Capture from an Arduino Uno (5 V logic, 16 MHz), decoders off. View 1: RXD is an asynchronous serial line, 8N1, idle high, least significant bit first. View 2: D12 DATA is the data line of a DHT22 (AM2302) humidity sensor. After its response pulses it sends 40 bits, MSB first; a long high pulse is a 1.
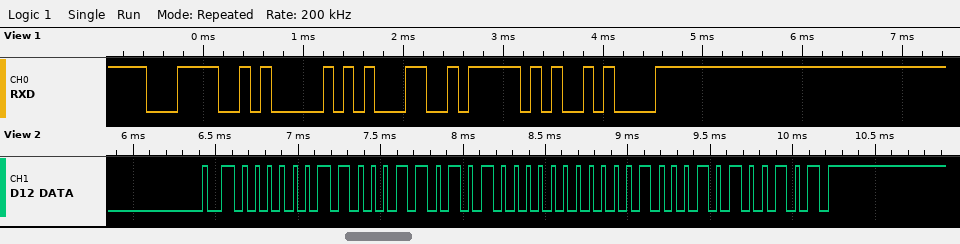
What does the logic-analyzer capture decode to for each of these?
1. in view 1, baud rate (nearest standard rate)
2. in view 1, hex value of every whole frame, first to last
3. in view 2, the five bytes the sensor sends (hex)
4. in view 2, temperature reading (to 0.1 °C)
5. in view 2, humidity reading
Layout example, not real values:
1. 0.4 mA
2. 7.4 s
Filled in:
1. 9600 baud
2. 0x3C 0x41 0x31 0x5F 0x0A
3. 03 1A 80 08 A5
4. -0.8 °C
5. 79.4 %
